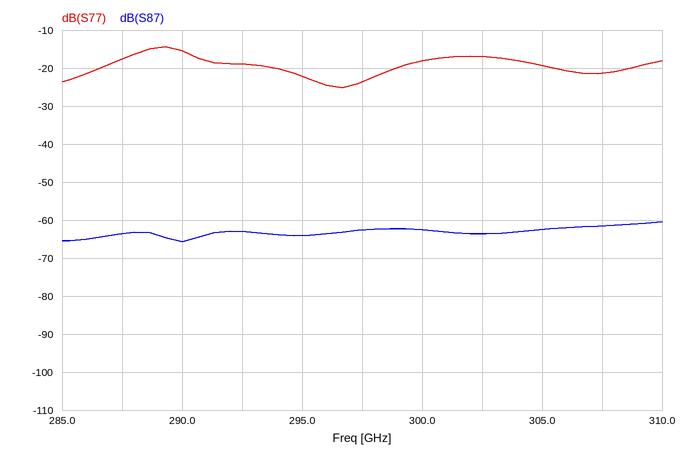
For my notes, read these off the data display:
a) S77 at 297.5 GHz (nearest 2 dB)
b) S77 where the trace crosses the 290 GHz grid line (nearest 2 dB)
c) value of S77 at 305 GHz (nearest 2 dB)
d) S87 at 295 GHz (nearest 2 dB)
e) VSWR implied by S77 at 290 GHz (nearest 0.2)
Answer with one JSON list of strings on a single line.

["-24 dB", "-16 dB", "-20 dB", "-64 dB", "1.4"]
